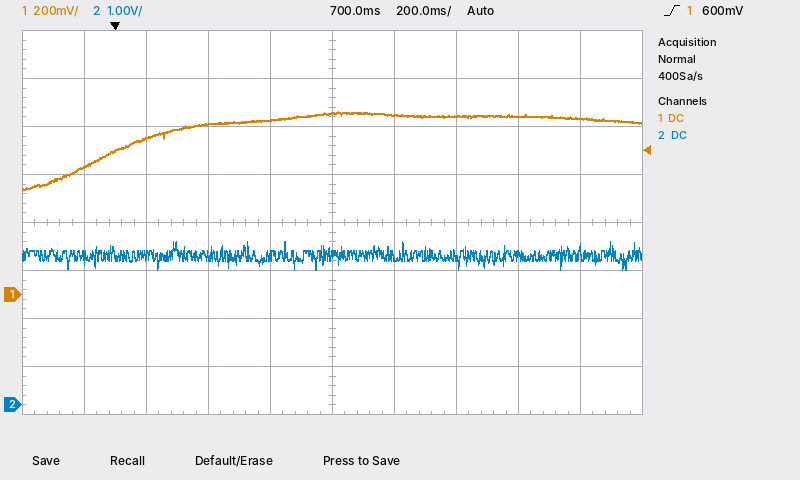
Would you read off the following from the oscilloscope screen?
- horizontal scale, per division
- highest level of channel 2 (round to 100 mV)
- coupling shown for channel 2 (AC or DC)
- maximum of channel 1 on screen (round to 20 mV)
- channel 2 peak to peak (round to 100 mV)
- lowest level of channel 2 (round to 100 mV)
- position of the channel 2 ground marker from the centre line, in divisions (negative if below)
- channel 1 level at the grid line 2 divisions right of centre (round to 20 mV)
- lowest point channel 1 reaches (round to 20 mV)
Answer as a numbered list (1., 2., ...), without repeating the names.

1. 200 ms
2. 3.4 V
3. DC
4. 760 mV
5. 600 mV
6. 2.8 V
7. -3.8 div
8. 740 mV
9. 440 mV
